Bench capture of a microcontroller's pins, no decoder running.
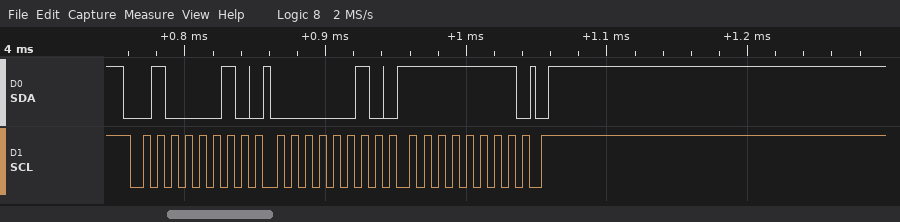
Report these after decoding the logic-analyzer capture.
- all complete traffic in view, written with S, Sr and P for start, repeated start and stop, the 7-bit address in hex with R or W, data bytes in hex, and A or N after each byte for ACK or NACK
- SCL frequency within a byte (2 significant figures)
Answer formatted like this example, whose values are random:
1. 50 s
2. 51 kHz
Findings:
1. S 21W A 02 A FF A P
2. 100 kHz
